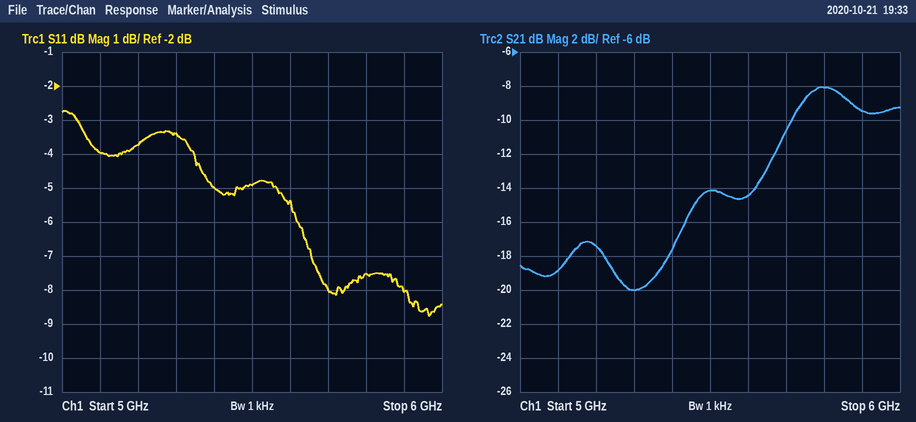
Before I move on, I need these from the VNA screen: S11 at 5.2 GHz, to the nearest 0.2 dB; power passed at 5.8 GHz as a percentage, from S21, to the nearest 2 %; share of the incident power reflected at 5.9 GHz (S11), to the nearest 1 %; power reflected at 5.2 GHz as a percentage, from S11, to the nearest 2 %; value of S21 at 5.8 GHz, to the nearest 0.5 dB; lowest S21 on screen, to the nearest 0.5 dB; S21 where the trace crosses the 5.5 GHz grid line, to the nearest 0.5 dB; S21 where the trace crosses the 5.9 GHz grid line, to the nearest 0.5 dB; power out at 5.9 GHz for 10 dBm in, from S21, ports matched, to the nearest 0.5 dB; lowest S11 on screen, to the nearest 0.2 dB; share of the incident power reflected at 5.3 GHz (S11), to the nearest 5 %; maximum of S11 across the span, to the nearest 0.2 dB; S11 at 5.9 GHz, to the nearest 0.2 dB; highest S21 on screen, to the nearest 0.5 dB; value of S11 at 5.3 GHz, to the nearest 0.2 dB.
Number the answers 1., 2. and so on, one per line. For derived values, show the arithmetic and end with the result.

1. -3.8 dB
2. 10^(-8/10) ≈ 16 %
3. 10^(-8/10) ≈ 16 %
4. 10^(-3.8/10) ≈ 42 %
5. -8.0 dB
6. -20.0 dB
7. -14.0 dB
8. -9.5 dB
9. 10 dBm + (-9.5 dB) = 0.5 dBm
10. -8.8 dB
11. 10^(-3.4/10) ≈ 45.7 %, so 45 % to the nearest 5 %
12. -2.8 dB
13. -8.0 dB
14. -8.0 dB
15. -3.4 dB
